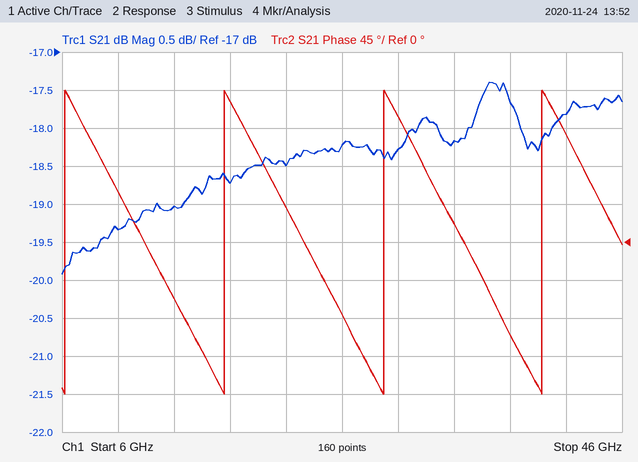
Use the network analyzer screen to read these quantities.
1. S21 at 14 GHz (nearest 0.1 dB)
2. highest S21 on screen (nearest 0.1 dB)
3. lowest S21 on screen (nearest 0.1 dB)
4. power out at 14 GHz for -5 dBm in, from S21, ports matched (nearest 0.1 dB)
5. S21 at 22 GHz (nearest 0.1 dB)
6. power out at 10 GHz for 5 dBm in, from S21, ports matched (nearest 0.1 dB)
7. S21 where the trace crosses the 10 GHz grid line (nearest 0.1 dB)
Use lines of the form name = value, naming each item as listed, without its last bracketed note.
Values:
S21 at 14 GHz = -19.0 dB
highest S21 on screen = -17.4 dB
lowest S21 on screen = -19.9 dB
power out at 14 GHz for -5 dBm in, from S21, ports matched = -24.0 dBm
S21 at 22 GHz = -18.5 dB
power out at 10 GHz for 5 dBm in, from S21, ports matched = -14.3 dBm
S21 where the trace crosses the 10 GHz grid line = -19.3 dB
